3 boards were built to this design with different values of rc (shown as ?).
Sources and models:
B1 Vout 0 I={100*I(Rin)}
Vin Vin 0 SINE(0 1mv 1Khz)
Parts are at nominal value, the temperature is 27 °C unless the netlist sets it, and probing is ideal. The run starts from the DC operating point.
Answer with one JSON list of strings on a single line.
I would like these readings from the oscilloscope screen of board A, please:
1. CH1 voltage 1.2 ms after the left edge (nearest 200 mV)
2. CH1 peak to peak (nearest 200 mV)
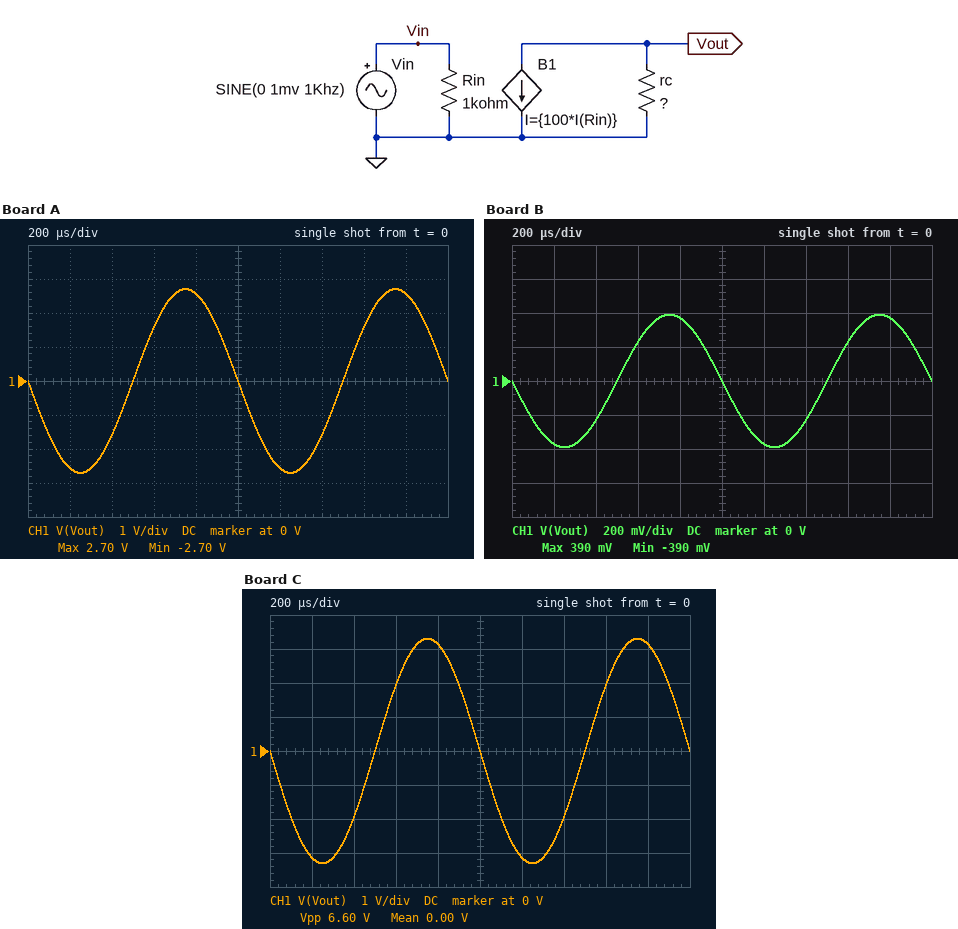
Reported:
["-2.6 V", "5.4 V"]
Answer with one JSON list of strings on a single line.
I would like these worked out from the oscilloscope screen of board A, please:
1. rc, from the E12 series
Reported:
["27 kΩ"]
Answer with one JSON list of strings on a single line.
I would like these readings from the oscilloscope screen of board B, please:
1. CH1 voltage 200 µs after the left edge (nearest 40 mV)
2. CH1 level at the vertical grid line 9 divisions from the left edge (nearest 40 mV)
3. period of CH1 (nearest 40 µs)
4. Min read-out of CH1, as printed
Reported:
["-360 mV", "360 mV", "1.00 ms", "-390 mV"]
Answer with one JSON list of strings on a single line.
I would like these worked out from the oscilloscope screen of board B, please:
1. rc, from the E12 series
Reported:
["3.9 kΩ"]
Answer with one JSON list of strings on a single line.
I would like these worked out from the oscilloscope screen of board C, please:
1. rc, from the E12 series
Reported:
["33 kΩ"]
